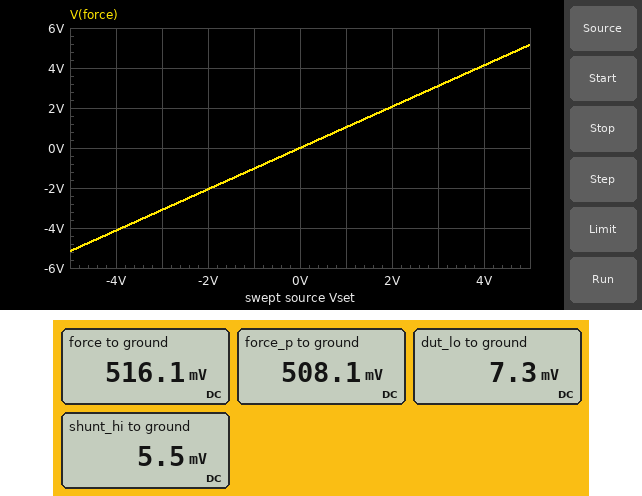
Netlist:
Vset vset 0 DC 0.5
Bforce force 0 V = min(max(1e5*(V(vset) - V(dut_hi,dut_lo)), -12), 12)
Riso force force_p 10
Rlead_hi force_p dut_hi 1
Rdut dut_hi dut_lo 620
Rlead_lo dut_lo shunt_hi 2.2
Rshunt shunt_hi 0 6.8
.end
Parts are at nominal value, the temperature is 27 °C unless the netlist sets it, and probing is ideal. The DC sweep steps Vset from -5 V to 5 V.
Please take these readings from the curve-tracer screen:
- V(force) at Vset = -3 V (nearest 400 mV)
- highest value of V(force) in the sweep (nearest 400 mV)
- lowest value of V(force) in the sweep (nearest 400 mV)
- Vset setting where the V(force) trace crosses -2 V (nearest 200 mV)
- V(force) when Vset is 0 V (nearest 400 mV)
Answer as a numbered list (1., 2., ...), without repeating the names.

1. -3.2 V
2. 5.2 V
3. -5.2 V
4. -2.0 V
5. 0 V
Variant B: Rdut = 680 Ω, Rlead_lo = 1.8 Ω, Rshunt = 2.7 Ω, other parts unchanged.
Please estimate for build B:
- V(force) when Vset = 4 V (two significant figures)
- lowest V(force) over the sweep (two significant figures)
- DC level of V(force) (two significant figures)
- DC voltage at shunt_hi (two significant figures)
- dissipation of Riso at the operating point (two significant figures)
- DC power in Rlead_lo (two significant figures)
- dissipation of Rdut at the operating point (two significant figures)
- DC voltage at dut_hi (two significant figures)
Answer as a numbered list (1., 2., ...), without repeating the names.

1. 4.1 V
2. -5.1 V
3. 510 mV
4. 2.0 mV
5. 5.4 µW
6. 970 nW
7. 370 µW
8. 500 mV
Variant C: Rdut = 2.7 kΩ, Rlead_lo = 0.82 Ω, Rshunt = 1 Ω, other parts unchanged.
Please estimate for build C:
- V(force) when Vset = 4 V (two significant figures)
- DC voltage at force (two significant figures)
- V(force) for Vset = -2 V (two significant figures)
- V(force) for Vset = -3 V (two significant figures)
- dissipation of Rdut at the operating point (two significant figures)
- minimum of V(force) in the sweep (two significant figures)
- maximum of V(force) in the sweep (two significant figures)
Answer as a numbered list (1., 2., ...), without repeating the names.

1. 4.0 V
2. 500 mV
3. -2.0 V
4. -3.0 V
5. 93 µW
6. -5.0 V
7. 5.0 V
